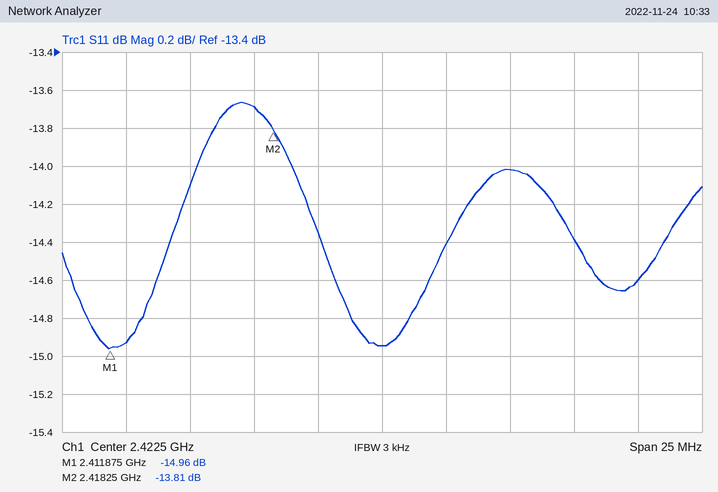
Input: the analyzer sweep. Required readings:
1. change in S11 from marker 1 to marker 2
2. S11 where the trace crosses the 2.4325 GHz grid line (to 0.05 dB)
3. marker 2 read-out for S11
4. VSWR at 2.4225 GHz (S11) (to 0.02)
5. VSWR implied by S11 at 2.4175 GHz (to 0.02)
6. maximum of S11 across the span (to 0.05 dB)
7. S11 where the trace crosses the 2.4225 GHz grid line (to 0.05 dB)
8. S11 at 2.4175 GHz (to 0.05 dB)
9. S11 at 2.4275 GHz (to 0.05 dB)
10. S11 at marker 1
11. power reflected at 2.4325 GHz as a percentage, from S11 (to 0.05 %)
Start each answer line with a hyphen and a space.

- 1.15 dB
- -14.60 dB
- -13.81 dB
- 1.44
- 1.52
- -13.65 dB
- -14.95 dB
- -13.70 dB
- -14.00 dB
- -14.96 dB
- 3.45 %
